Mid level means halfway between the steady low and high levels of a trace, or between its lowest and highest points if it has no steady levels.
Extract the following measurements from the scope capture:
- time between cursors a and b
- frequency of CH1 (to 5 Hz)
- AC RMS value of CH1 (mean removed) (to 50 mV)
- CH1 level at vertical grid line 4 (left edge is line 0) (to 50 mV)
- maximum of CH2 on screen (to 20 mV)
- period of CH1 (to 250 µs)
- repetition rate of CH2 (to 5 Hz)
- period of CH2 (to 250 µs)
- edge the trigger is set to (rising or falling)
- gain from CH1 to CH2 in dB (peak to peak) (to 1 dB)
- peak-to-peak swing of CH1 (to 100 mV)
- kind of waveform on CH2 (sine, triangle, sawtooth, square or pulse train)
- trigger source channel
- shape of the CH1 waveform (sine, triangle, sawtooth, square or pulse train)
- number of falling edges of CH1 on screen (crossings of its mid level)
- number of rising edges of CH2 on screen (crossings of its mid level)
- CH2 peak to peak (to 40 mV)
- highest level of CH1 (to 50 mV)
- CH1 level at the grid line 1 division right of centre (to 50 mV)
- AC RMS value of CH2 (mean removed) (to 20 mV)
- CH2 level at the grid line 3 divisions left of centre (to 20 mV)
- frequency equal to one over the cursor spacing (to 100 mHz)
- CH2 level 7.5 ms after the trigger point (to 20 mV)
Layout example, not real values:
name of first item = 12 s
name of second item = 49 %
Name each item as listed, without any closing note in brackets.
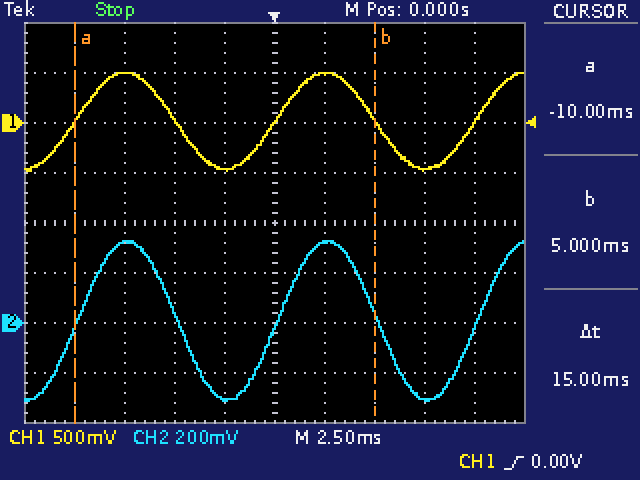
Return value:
time between cursors a and b = 15 ms
frequency of CH1 = 100 Hz
AC RMS value of CH1 (mean removed) = 350 mV
CH1 level at vertical grid line 4 (left edge is line 0) = -450 mV
maximum of CH2 on screen = 320 mV
period of CH1 = 10.00 ms
repetition rate of CH2 = 100 Hz
period of CH2 = 10.00 ms
edge the trigger is set to = rising
gain from CH1 to CH2 in dB (peak to peak) = -4 dB
peak-to-peak swing of CH1 = 1.00 V
kind of waveform on CH2 = sine
trigger source channel = CH1
shape of the CH1 waveform = sine
number of falling edges of CH1 on screen = 2
number of rising edges of CH2 on screen = 3
CH2 peak to peak = 640 mV
highest level of CH1 = 500 mV
CH1 level at the grid line 1 division right of centre = 500 mV
AC RMS value of CH2 (mean removed) = 220 mV
CH2 level at the grid line 3 divisions left of centre = 320 mV
frequency equal to one over the cursor spacing = 66.7 Hz
CH2 level 7.5 ms after the trigger point = -300 mV
